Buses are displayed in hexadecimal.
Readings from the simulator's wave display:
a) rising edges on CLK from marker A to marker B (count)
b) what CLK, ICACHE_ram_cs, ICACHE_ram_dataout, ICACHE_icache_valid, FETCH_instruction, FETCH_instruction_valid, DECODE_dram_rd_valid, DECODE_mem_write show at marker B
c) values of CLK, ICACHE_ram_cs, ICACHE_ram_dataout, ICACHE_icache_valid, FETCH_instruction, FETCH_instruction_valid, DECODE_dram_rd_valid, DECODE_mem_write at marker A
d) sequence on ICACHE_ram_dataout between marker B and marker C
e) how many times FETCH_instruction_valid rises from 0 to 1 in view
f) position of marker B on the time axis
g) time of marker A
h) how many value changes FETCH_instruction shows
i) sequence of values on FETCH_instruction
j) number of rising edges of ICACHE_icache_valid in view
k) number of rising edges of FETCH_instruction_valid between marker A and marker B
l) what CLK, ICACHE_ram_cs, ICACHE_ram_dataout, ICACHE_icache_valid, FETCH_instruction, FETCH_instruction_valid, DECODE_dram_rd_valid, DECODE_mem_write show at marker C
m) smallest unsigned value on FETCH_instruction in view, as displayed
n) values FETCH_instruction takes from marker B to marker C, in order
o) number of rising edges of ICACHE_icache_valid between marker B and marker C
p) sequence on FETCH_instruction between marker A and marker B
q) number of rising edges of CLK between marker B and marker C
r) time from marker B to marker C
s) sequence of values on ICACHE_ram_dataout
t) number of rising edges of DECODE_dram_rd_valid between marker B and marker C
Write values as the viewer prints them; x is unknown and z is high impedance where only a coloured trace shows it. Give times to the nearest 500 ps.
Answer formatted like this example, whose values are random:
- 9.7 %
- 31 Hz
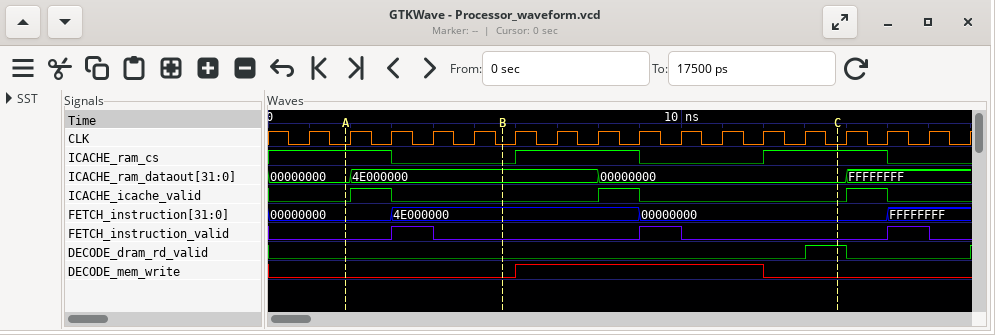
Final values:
- 4
- CLK=0, ICACHE_ram_cs=0, ICACHE_ram_dataout=4E000000, ICACHE_icache_valid=0, FETCH_instruction=4E000000, FETCH_instruction_valid=0, DECODE_dram_rd_valid=0, DECODE_mem_write=0
- CLK=0, ICACHE_ram_cs=1, ICACHE_ram_dataout=00000000, ICACHE_icache_valid=0, FETCH_instruction=00000000, FETCH_instruction_valid=0, DECODE_dram_rd_valid=0, DECODE_mem_write=0
- 4E000000, 00000000
- 3
- 5500 ps
- 2000 ps
- 3
- 00000000, 4E000000, 00000000, FFFFFFFF
- 3
- 1
- CLK=0, ICACHE_ram_cs=1, ICACHE_ram_dataout=00000000, ICACHE_icache_valid=0, FETCH_instruction=00000000, FETCH_instruction_valid=0, DECODE_dram_rd_valid=1, DECODE_mem_write=0
- 00000000
- 4E000000, 00000000
- 1
- 00000000, 4E000000
- 8
- 8000 ps
- 00000000, 4E000000, 00000000, FFFFFFFF
- 1
